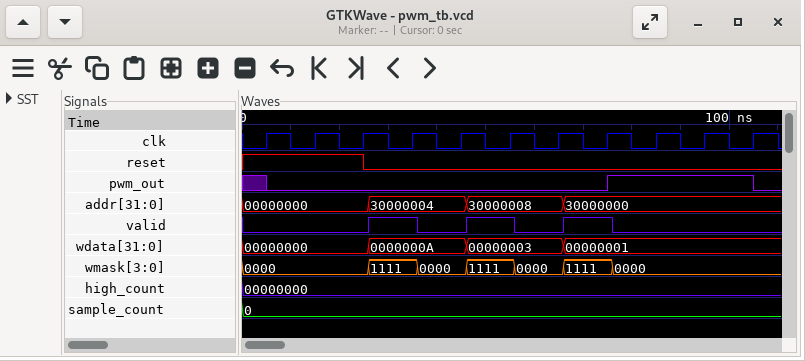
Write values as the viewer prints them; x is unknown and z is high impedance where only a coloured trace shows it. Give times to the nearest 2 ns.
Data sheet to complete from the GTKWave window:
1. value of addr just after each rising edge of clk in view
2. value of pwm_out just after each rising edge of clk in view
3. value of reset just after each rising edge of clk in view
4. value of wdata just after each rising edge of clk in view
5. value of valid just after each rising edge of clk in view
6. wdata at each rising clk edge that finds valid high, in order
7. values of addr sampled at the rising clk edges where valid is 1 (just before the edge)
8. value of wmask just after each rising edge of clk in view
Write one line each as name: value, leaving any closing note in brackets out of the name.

value of addr just after each rising edge of clk in view: 00000000, 00000000, 00000000, 30000004, 30000004, 30000008, 30000008, 30000000, 30000000, 30000000, 30000000
value of pwm_out just after each rising edge of clk in view: 0 0 0 0 0 0 0 1 1 1 0
value of reset just after each rising edge of clk in view: 1 1 0 0 0 0 0 0 0 0 0
value of wdata just after each rising edge of clk in view: 00000000, 00000000, 00000000, 0000000A, 0000000A, 00000003, 00000003, 00000001, 00000001, 00000001, 00000001
value of valid just after each rising edge of clk in view: 0 0 0 1 0 1 0 1 0 0 0
wdata at each rising clk edge that finds valid high, in order: 0000000A, 00000003, 00000001
values of addr sampled at the rising clk edges where valid is 1: 30000004, 30000008, 30000000
value of wmask just after each rising edge of clk in view: 0000, 0000, 0000, 1111, 0000, 1111, 0000, 1111, 0000, 0000, 0000
